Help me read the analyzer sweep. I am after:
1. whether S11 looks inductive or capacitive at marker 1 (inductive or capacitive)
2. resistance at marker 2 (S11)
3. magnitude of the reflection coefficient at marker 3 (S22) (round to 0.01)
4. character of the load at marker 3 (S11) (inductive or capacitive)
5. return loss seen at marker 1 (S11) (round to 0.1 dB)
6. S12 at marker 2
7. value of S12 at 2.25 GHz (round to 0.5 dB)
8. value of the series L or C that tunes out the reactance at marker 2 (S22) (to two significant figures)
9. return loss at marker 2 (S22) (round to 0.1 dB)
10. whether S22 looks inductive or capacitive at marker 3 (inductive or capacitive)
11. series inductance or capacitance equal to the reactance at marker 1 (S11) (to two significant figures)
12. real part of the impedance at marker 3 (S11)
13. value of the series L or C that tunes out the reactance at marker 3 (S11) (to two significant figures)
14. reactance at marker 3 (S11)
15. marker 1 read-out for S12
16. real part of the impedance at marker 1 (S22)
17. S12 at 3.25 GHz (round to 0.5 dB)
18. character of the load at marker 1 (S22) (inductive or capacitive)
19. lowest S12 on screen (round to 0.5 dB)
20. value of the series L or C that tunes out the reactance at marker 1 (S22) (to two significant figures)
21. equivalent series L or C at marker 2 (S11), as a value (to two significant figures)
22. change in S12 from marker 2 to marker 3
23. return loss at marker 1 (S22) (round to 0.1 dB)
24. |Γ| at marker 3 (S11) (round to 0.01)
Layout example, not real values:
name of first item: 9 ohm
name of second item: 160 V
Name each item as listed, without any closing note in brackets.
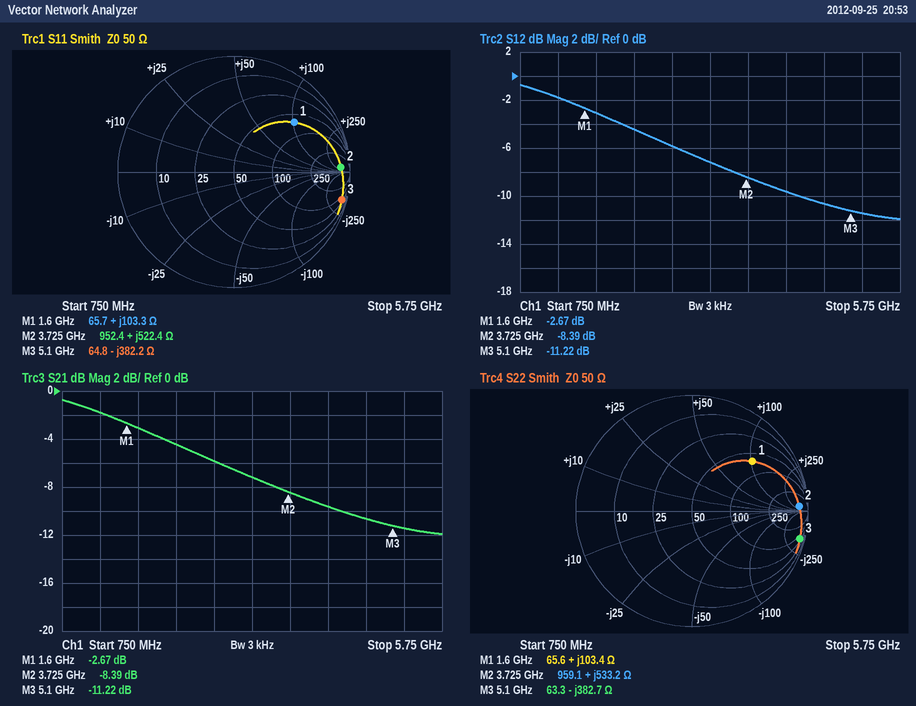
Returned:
whether S11 looks inductive or capacitive at marker 1: inductive
resistance at marker 2: 952.4 Ω
magnitude of the reflection coefficient at marker 3 (S22): 0.96
character of the load at marker 3 (S11): capacitive
return loss seen at marker 1 (S11): 3.4 dB
S12 at marker 2: -8.39 dB
value of S12 at 2.25 GHz: -4.5 dB
value of the series L or C that tunes out the reactance at marker 2 (S22): 80 fF
return loss at marker 2 (S22): 0.7 dB
whether S22 looks inductive or capacitive at marker 3: capacitive
series inductance or capacitance equal to the reactance at marker 1 (S11): 10 nH
real part of the impedance at marker 3: 64.8 Ω
value of the series L or C that tunes out the reactance at marker 3 (S11): 12 nH
reactance at marker 3: -382.2 Ω
marker 1 read-out for S12: -2.67 dB
real part of the impedance at marker 1: 65.6 Ω
S12 at 3.25 GHz: -7.0 dB
character of the load at marker 1 (S22): inductive
lowest S12 on screen: -12.0 dB
value of the series L or C that tunes out the reactance at marker 1 (S22): 960 fF
equivalent series L or C at marker 2 (S11), as a value: 22 nH
change in S12 from marker 2 to marker 3: -2.83 dB
return loss at marker 1 (S22): 3.4 dB
|Γ| at marker 3 (S11): 0.96
